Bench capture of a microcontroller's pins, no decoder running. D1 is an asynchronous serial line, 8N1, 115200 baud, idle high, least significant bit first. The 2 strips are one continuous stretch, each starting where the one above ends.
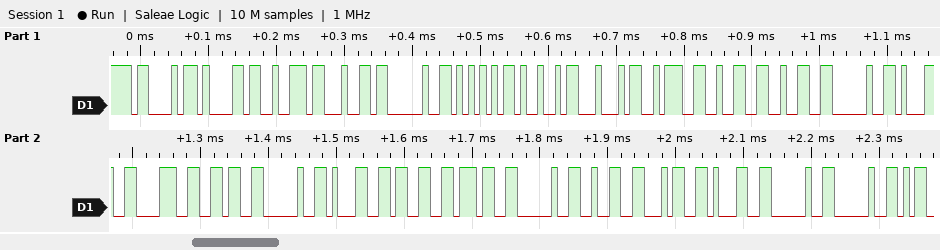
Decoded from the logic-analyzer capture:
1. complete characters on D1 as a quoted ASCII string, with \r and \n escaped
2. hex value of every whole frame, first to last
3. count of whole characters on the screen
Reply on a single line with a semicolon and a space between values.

"Card UID:22 186 137 241  "; 43 61 72 64 20 55 49 44 3A 32 32 20 31 38 36 20 31 33 37 20 32 34 31 20 20; 25
